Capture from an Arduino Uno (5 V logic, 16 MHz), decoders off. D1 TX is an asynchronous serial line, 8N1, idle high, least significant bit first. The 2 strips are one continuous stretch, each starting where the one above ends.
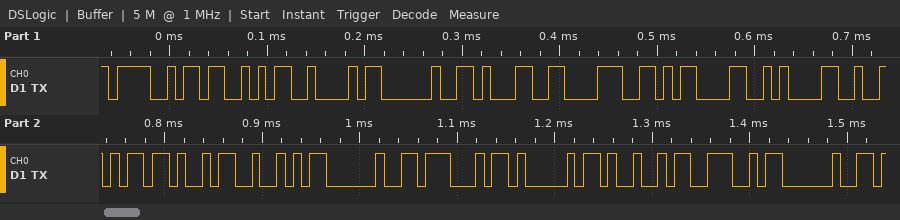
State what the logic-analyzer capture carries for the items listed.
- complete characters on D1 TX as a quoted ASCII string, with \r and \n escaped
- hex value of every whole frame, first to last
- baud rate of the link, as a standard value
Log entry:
"OSB 18\r\nRKR GAIN "
4F 53 42 20 31 38 0D 0A 52 4B 52 20 47 41 49 4E 20
115200 baud
